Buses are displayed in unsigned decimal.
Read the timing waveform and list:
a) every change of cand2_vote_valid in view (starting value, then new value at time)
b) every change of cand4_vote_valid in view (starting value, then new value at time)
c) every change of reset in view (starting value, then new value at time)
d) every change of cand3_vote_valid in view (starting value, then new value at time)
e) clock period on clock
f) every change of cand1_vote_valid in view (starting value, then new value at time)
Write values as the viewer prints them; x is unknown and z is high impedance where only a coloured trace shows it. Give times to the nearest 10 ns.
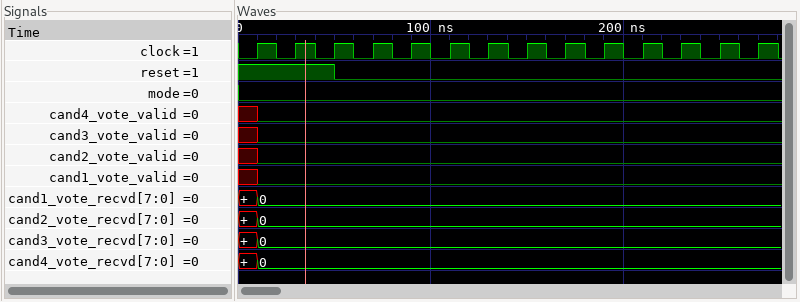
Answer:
x, 0 at 10 ns
x, 0 at 10 ns
1, 0 at 50 ns
x, 0 at 10 ns
20 ns
x, 0 at 10 ns
